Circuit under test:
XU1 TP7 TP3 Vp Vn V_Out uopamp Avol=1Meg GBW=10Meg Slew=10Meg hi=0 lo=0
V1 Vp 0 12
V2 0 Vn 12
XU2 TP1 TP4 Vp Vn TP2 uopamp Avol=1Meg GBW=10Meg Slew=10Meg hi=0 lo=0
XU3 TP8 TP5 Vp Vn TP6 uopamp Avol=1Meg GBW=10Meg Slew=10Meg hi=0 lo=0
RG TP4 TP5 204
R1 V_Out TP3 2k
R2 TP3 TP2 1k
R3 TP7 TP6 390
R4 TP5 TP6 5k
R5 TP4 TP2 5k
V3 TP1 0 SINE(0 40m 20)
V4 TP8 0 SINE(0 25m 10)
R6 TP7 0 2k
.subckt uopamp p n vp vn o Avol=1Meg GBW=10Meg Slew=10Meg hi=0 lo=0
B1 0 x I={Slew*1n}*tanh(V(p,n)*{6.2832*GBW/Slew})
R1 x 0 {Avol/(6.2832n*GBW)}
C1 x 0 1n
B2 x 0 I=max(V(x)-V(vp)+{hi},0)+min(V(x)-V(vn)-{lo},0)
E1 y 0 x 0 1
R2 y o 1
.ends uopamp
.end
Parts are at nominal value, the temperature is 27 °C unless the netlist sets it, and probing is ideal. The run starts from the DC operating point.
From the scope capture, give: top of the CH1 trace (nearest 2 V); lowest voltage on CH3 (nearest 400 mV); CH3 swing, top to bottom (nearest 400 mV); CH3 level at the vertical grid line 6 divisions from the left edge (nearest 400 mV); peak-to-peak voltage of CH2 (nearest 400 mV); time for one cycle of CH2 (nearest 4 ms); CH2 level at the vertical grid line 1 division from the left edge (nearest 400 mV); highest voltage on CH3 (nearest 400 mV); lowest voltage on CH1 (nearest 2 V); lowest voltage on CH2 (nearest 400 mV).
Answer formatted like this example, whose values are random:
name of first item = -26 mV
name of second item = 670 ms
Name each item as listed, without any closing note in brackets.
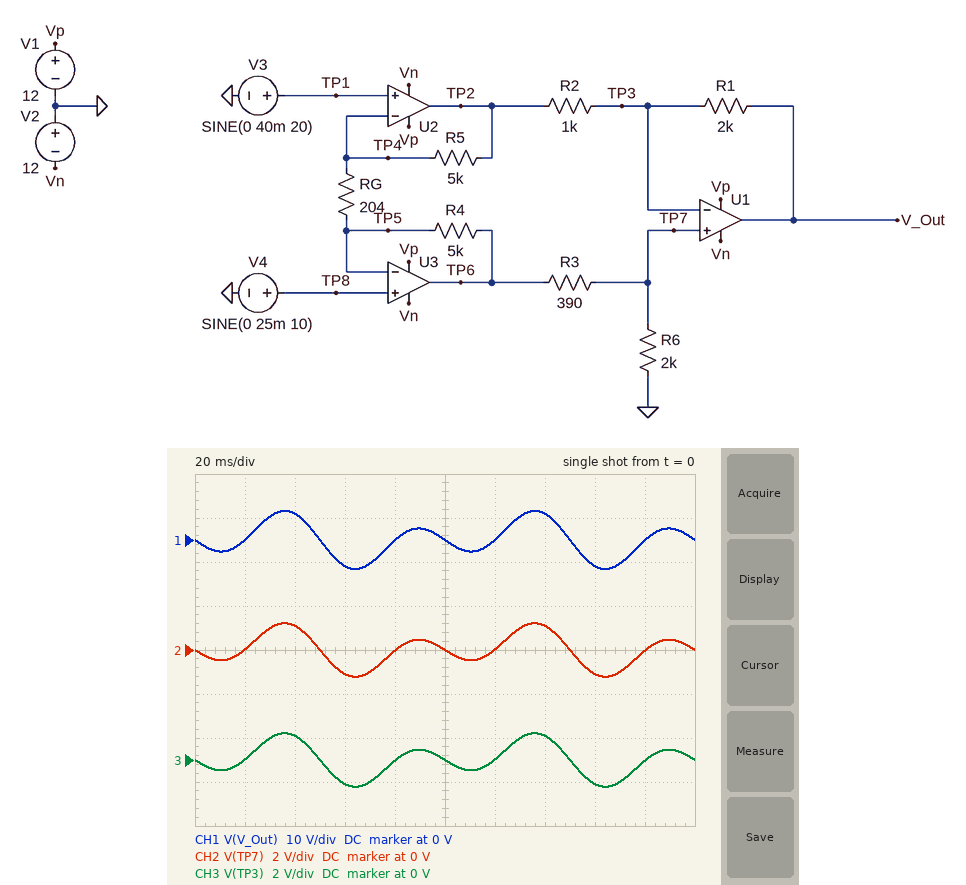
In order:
top of the CH1 trace = 6 V
lowest voltage on CH3 = -1.2 V
CH3 swing, top to bottom = 2.4 V
CH3 level at the vertical grid line 6 divisions from the left edge = 0 V
peak-to-peak voltage of CH2 = 2.4 V
time for one cycle of CH2 = 100 ms
CH2 level at the vertical grid line 1 division from the left edge = 0 V
highest voltage on CH3 = 1.2 V
lowest voltage on CH1 = -6 V
lowest voltage on CH2 = -1.2 V
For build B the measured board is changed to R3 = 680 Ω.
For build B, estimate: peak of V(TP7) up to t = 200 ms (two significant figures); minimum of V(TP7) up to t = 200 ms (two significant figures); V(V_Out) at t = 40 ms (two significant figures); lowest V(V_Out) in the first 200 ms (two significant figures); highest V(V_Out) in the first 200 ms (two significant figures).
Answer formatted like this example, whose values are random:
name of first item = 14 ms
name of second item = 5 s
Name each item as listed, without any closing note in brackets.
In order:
peak of V(TP7) up to t = 200 ms = 1.1 V
minimum of V(TP7) up to t = 200 ms = -1.1 V
V(V_Out) at t = 40 ms = 5.6 V
lowest V(V_Out) in the first 200 ms = -6.2 V
highest V(V_Out) in the first 200 ms = 6.2 V
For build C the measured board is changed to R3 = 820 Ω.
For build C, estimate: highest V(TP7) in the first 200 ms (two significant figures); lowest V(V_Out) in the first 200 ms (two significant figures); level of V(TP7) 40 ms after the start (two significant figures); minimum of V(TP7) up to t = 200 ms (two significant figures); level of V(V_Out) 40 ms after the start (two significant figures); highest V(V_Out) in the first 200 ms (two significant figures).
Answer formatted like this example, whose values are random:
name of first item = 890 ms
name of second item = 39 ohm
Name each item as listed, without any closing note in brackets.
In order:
highest V(TP7) in the first 200 ms = 1.0 V
lowest V(V_Out) in the first 200 ms = -6.0 V
level of V(TP7) 40 ms after the start = 930 mV
minimum of V(TP7) up to t = 200 ms = -1.0 V
level of V(V_Out) 40 ms after the start = 5.4 V
highest V(V_Out) in the first 200 ms = 6.0 V
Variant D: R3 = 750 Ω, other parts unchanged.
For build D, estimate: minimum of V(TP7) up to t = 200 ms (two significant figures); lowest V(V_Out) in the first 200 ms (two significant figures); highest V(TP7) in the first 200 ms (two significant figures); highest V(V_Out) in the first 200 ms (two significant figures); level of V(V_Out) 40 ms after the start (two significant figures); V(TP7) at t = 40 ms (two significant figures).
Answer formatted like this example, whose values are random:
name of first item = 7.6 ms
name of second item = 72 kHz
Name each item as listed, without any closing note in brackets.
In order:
minimum of V(TP7) up to t = 200 ms = -1.1 V
lowest V(V_Out) in the first 200 ms = -6.1 V
highest V(TP7) in the first 200 ms = 1.1 V
highest V(V_Out) in the first 200 ms = 6.1 V
level of V(V_Out) 40 ms after the start = 5.5 V
V(TP7) at t = 40 ms = 950 mV
